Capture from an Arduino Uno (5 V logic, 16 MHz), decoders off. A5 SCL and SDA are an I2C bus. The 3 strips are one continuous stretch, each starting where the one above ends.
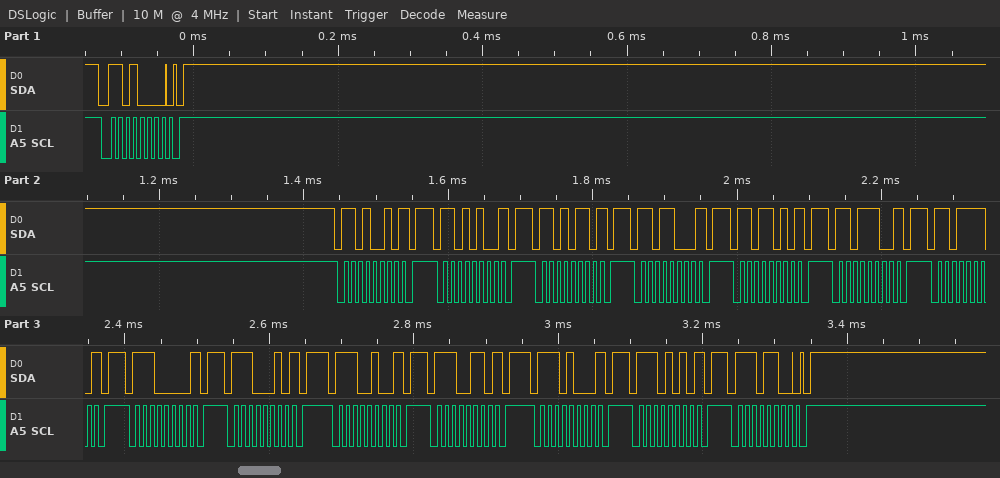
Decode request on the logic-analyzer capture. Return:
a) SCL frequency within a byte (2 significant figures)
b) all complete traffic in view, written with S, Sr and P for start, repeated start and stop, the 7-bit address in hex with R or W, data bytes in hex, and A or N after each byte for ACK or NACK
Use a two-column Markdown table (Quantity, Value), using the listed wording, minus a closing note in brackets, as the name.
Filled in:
| Quantity | Value |
|---|---|
| SCL frequency within a byte | 100 kHz |
| all complete traffic in view, written with S, Sr and P for start, repeated start and stop, the 7-bit address in hex with R or W, data bytes in hex, and A or N after each byte for ACK or NACK | S 68W A P S 69W N P S 6AW N P S 6BW N P S 6CW N P S 6DW N P S 6EW N P S 6FW N P S 70W N P S 71W N P S 72W N P S 73W N P S 74W N P S 75W N P S 76W A P |
